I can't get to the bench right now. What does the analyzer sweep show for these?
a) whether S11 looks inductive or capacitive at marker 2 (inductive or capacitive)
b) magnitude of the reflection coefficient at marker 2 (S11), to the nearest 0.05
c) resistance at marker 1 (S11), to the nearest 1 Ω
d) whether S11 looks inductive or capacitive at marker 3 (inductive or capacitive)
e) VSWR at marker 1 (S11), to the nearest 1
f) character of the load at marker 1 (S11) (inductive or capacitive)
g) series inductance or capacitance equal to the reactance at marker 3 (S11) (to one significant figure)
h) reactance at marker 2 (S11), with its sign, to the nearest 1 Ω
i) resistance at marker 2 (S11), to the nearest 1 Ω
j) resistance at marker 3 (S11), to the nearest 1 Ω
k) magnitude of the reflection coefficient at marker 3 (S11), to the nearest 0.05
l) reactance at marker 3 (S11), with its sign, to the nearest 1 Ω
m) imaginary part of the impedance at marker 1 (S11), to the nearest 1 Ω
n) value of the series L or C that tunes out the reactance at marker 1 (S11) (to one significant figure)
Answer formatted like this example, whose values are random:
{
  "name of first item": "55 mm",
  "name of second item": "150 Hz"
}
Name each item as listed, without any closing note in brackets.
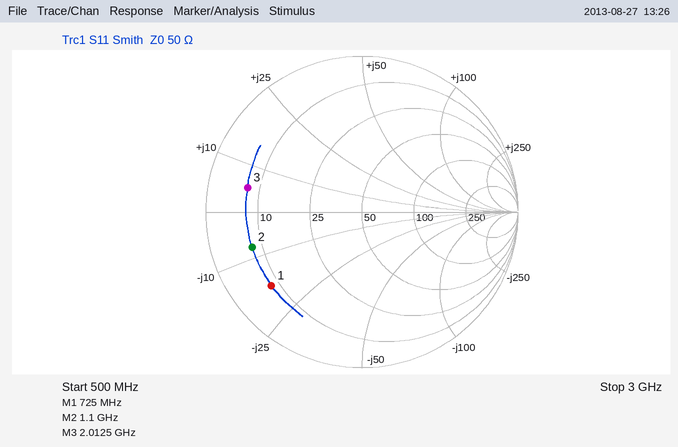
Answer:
{
  "whether S11 looks inductive or capacitive at marker 2": "capacitive",
  "magnitude of the reflection coefficient at marker 2 (S11), to the nearest 0.05": "0.75",
  "resistance at marker 1 (S11), to the nearest 1 Ω": "8 Ω",
  "whether S11 looks inductive or capacitive at marker 3": "inductive",
  "VSWR at marker 1 (S11), to the nearest 1": "7",
  "character of the load at marker 1 (S11)": "capacitive",
  "series inductance or capacitance equal to the reactance at marker 3 (S11)": "400 pH",
  "reactance at marker 2 (S11), with its sign, to the nearest 1 Ω": "-8 Ω",
  "resistance at marker 2 (S11), to the nearest 1 Ω": "8 Ω",
  "resistance at marker 3 (S11), to the nearest 1 Ω": "7 Ω",
  "magnitude of the reflection coefficient at marker 3 (S11), to the nearest 0.05": "0.75",
  "reactance at marker 3 (S11), with its sign, to the nearest 1 Ω": "+5 Ω",
  "imaginary part of the impedance at marker 1 (S11), to the nearest 1 Ω": "-17 Ω",
  "value of the series L or C that tunes out the reactance at marker 1 (S11)": "4 nH"
}
